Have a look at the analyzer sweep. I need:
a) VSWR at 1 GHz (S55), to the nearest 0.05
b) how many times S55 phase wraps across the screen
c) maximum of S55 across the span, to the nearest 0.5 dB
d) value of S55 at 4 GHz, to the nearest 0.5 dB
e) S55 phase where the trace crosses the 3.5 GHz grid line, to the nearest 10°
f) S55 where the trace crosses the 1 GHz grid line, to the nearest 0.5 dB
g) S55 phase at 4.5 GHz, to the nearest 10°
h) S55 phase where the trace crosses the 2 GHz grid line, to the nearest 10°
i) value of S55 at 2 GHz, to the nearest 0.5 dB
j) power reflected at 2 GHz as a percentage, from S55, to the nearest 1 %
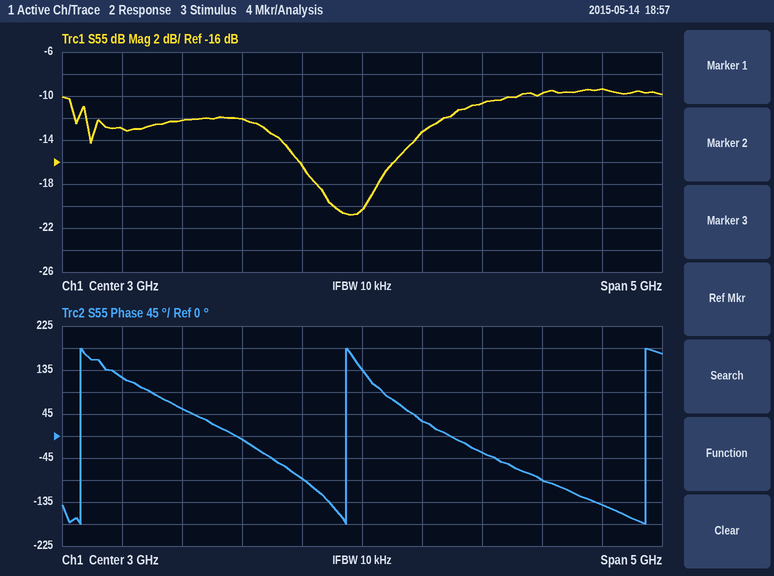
1.60
3
-9.5 dB
-10.5 dB
30°
-13.0 dB
-90°
-10°
-12.0 dB
6 %
